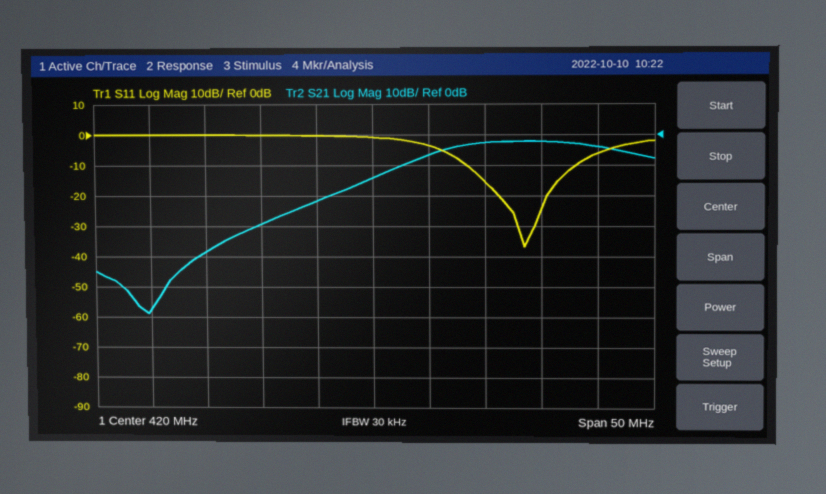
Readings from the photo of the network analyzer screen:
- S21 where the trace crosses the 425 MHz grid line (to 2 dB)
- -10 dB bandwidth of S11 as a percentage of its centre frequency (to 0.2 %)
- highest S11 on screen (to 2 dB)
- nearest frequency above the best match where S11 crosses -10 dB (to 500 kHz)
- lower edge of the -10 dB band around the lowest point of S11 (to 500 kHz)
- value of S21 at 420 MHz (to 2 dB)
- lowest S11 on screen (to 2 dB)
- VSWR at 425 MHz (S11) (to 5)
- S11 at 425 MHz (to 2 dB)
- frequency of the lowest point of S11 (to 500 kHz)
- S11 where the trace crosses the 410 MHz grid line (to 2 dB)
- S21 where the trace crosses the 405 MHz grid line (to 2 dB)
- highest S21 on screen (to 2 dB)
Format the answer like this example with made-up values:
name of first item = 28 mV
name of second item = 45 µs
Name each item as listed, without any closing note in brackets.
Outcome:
S21 where the trace crosses the 425 MHz grid line = -6 dB
-10 dB bandwidth of S11 as a percentage of its centre frequency = 2.2 %
highest S11 on screen = 0 dB
nearest frequency above the best match where S11 crosses -10 dB = 438.0 MHz
lower edge of the -10 dB band around the lowest point of S11 = 428.5 MHz
value of S21 at 420 MHz = -14 dB
lowest S11 on screen = -36 dB
VSWR at 425 MHz (S11) = 5
S11 at 425 MHz = -4 dB
frequency of the lowest point of S11 = 433.5 MHz
S11 where the trace crosses the 410 MHz grid line = 0 dB
S21 where the trace crosses the 405 MHz grid line = -38 dB
highest S21 on screen = -2 dB
